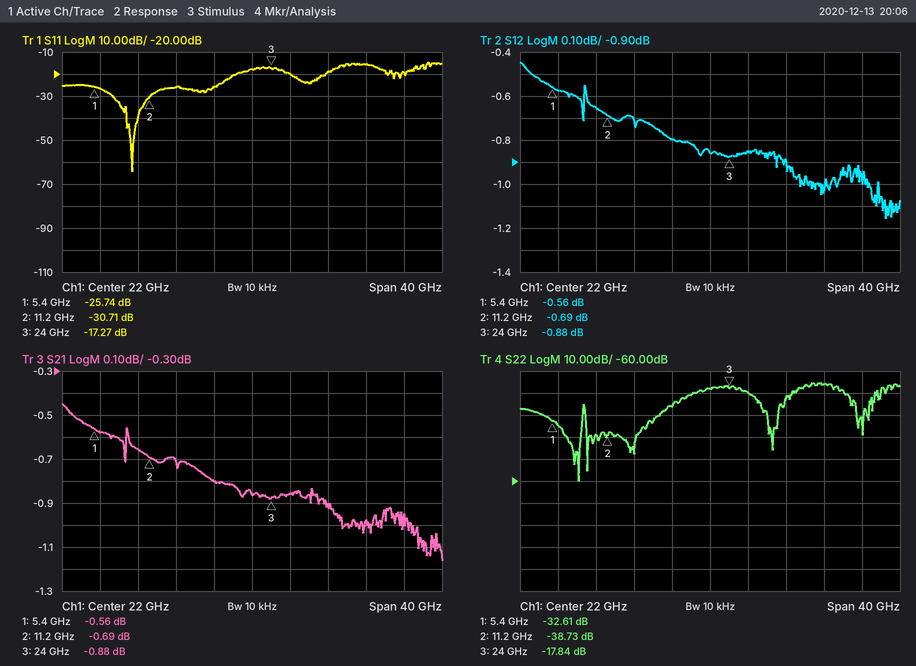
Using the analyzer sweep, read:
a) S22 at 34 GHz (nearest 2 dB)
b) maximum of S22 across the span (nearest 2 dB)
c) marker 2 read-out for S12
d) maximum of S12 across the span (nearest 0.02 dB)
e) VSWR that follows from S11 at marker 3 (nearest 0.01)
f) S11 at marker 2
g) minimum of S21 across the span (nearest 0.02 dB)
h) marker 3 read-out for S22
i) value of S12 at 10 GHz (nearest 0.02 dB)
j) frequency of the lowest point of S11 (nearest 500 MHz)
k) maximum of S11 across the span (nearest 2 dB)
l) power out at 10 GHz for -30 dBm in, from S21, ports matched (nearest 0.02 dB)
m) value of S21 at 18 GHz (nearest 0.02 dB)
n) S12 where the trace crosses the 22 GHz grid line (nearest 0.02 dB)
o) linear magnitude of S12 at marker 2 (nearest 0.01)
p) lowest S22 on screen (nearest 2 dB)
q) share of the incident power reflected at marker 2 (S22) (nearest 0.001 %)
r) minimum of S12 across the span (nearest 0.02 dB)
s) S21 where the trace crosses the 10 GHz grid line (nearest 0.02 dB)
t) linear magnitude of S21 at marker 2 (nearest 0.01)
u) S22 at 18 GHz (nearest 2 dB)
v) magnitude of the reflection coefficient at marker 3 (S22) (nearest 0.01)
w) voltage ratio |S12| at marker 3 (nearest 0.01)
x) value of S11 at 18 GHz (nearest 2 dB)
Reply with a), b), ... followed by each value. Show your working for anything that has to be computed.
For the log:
a) -16 dB
b) -16 dB
c) -0.69 dB
d) -0.44 dB
e) (1 + 0.1369)/(1 − 0.1369) ≈ 1.32
f) -30.71 dB
g) -1.16 dB
h) -17.84 dB
i) -0.66 dB
j) 9.5 GHz
k) -14 dB
l) -30 dBm + (-0.66 dB) = -30.66 dBm
m) -0.80 dB
n) -0.86 dB
o) 10^(-0.69/20) ≈ 0.92
p) -60 dB
q) 10^(-38.73/10) ≈ 0.013 %
r) -1.16 dB
s) -0.66 dB
t) 10^(-0.69/20) ≈ 0.92
u) -26 dB
v) 10^(-17.84/20) ≈ 0.13
w) 10^(-0.88/20) ≈ 0.90
x) -26 dB
